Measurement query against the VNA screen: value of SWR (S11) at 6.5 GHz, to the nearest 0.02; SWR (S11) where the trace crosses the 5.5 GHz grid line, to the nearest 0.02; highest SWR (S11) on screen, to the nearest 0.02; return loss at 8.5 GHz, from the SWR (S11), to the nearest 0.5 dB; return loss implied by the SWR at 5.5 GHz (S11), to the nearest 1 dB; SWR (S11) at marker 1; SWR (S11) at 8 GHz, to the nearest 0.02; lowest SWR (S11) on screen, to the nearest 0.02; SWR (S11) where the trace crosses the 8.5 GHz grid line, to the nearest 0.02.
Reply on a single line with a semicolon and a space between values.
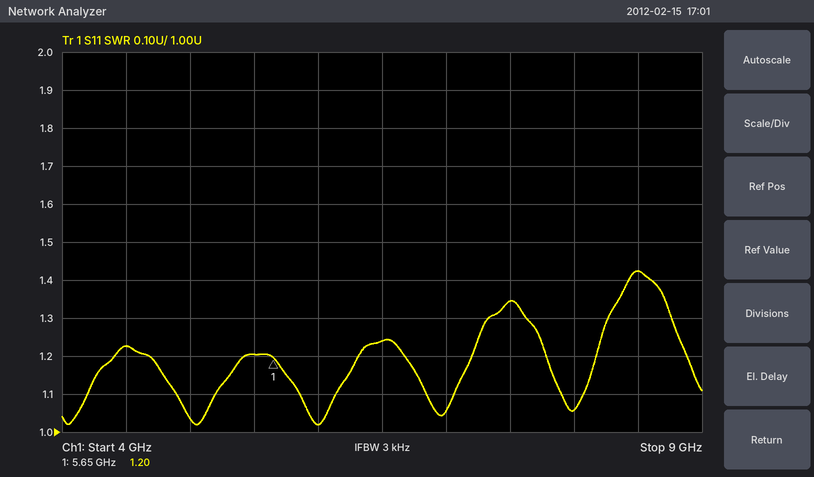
1.24; 1.20; 1.42; 15.0 dB; 21 dB; 1.20; 1.06; 1.02; 1.42
